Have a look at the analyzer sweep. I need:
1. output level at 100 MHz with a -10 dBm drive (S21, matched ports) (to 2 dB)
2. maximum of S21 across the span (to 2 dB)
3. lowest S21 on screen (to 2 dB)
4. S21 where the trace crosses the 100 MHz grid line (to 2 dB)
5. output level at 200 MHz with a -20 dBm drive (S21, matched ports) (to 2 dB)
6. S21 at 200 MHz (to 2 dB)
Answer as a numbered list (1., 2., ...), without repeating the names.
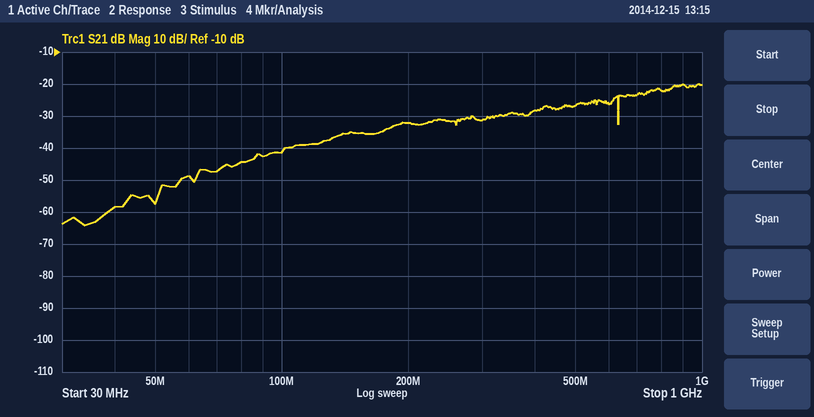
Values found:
1. -52 dBm
2. -20 dB
3. -64 dB
4. -42 dB
5. -52 dBm
6. -32 dB
